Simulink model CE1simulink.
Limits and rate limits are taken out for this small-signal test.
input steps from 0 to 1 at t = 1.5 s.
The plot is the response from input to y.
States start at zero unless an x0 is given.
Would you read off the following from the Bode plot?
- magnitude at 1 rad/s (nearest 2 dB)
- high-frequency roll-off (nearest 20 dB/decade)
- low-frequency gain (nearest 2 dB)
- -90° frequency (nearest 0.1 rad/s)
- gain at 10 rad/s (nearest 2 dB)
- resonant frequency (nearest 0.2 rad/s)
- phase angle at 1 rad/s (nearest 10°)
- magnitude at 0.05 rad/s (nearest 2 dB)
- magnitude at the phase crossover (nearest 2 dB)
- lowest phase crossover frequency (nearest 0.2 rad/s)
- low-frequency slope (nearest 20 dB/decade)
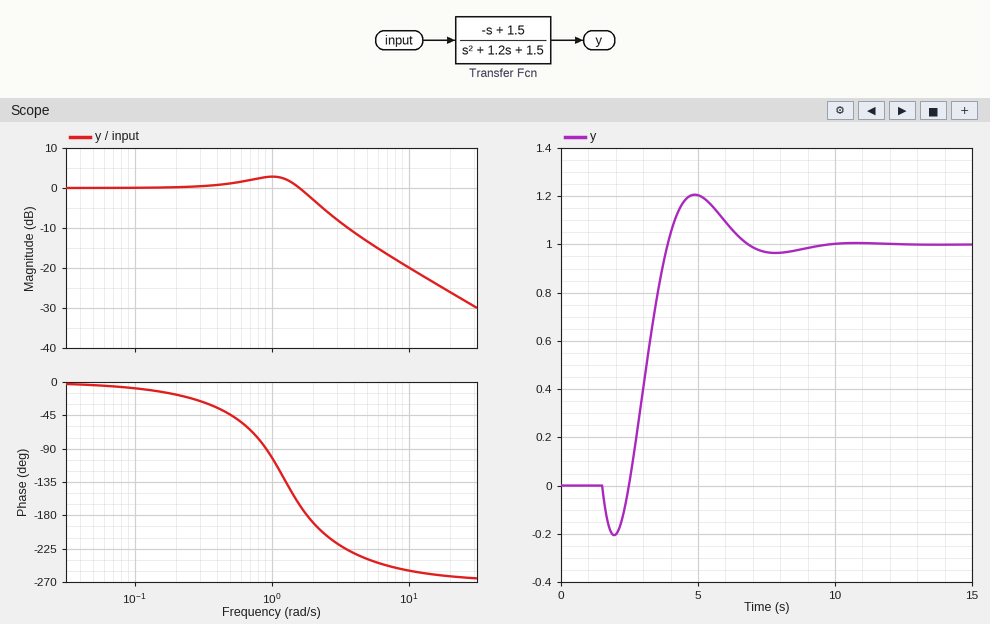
2 dB
-20 dB/decade
0 dB
0.9 rad/s
-20 dB
1.0 rad/s
-100°
0 dB
-2 dB
1.8 rad/s
0 dB/decade
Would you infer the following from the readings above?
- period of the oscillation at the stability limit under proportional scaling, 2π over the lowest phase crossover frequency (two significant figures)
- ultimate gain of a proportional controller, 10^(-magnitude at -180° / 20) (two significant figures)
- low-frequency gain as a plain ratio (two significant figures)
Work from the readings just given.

3.5 s
1.3
1.0
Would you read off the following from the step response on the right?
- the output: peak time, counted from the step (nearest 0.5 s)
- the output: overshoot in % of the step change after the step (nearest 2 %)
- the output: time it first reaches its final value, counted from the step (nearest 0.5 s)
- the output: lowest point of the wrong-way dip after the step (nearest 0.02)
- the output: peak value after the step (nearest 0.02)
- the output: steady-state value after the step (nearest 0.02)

3.5 s
20 %
2.5 s
-0.20
1.20
1.00
